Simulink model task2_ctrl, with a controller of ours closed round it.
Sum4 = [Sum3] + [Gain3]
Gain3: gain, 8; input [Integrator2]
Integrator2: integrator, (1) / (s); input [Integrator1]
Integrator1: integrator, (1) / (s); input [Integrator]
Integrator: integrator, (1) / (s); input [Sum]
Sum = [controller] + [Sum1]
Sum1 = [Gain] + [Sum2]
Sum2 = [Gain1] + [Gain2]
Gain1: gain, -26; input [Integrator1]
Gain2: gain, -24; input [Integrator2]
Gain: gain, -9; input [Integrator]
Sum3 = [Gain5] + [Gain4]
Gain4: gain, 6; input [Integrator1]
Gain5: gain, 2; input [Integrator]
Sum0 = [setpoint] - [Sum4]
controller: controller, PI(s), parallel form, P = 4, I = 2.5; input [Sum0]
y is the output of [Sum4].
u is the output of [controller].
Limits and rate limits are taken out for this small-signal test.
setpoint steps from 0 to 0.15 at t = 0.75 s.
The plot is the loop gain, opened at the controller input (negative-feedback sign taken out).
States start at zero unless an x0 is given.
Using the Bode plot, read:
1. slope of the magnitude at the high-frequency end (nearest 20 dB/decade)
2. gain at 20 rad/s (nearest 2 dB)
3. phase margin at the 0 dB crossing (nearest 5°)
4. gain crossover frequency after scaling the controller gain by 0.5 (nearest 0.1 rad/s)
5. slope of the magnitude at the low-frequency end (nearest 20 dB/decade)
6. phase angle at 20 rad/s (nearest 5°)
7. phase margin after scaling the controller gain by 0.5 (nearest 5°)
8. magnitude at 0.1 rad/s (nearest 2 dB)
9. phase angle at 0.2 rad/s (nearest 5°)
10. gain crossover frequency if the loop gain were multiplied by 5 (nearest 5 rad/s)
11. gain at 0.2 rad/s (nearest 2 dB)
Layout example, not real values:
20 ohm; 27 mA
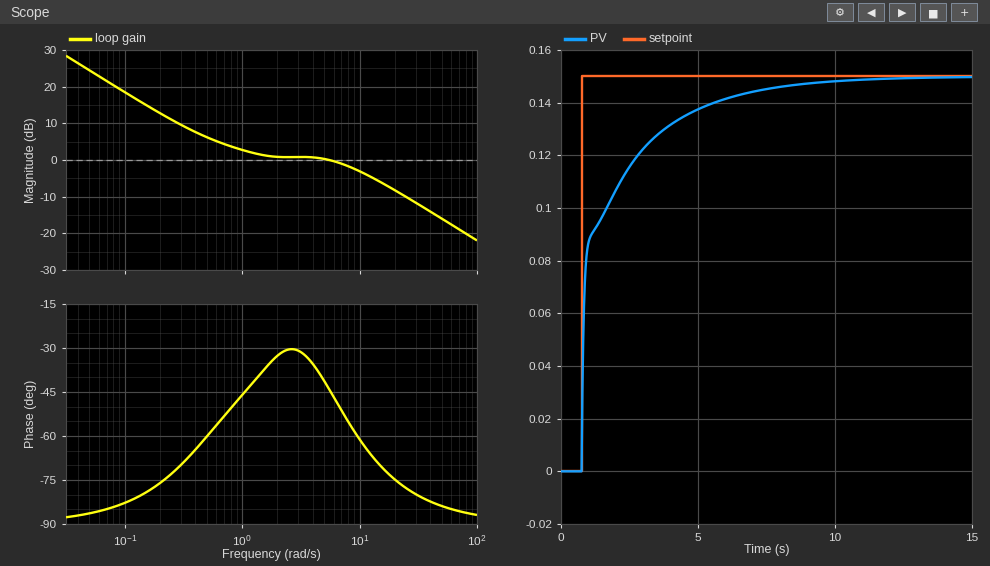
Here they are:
-20 dB/decade; -8 dB; 135°; 0.5 rad/s; -20 dB/decade; -75°; 120°; 18 dB; -75°; 40 rad/s; 12 dB
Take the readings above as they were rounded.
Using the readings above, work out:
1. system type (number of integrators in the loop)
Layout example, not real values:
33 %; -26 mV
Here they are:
1
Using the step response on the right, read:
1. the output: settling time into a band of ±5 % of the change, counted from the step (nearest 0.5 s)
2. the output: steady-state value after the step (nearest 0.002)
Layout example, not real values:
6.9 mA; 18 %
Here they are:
5.5 s; 0.150
